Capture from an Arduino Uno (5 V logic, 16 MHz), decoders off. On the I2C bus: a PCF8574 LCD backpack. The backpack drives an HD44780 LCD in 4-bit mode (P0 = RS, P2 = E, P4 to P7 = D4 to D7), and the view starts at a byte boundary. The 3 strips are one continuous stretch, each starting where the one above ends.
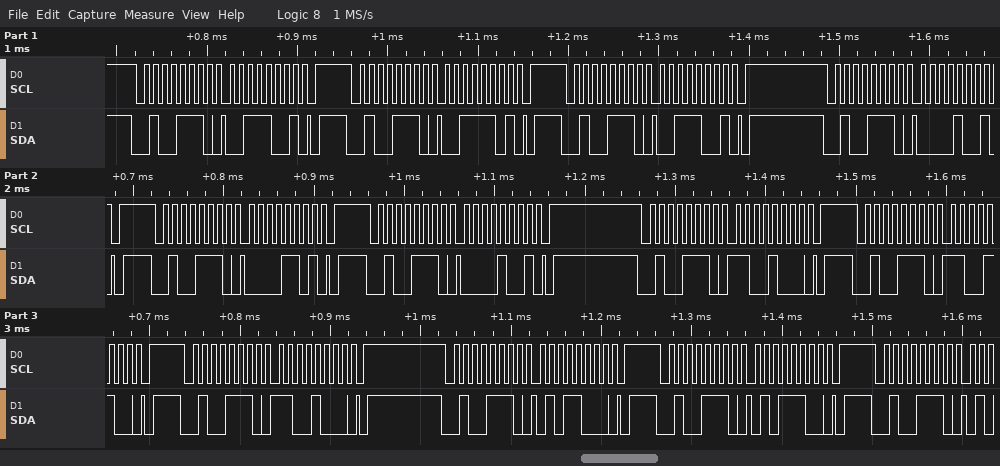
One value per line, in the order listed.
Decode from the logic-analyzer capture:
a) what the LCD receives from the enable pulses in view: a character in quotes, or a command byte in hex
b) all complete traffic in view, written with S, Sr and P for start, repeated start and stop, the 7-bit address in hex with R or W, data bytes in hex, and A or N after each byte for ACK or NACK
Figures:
'0'
S 27W A 39 A P S 27W A 3D A P S 27W A 39 A P S 27W A 09 A P S 27W A 0D A P S 27W A 09 A P S 27W A C8 A P S 27W A CC A P S 27W A C8 A P S 27W A 58 A P S 27W A 5C A P S 27W A
